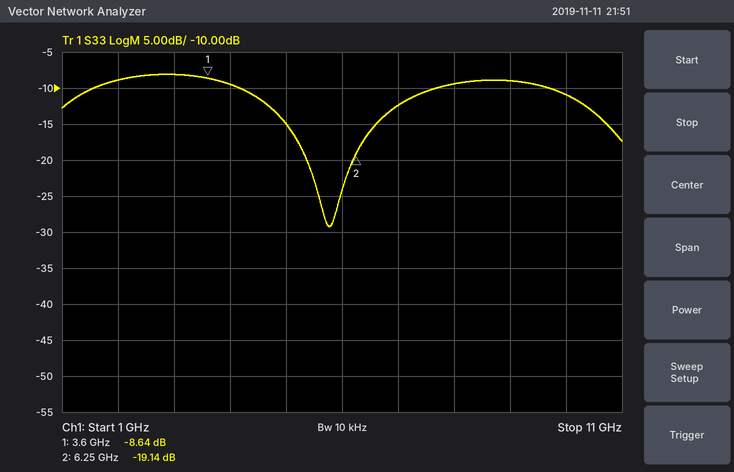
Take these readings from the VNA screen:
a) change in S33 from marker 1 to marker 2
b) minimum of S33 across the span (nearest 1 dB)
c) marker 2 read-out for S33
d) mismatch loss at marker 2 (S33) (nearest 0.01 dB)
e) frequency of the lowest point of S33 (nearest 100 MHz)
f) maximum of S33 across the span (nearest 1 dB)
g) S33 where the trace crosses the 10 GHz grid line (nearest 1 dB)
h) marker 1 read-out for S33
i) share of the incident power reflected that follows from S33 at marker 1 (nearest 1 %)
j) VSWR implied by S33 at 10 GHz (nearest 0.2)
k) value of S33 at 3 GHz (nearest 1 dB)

-10.50 dB
-29 dB
-19.14 dB
0.05 dB
5.8 GHz
-8 dB
-11 dB
-8.64 dB
14 %
1.8
-8 dB
